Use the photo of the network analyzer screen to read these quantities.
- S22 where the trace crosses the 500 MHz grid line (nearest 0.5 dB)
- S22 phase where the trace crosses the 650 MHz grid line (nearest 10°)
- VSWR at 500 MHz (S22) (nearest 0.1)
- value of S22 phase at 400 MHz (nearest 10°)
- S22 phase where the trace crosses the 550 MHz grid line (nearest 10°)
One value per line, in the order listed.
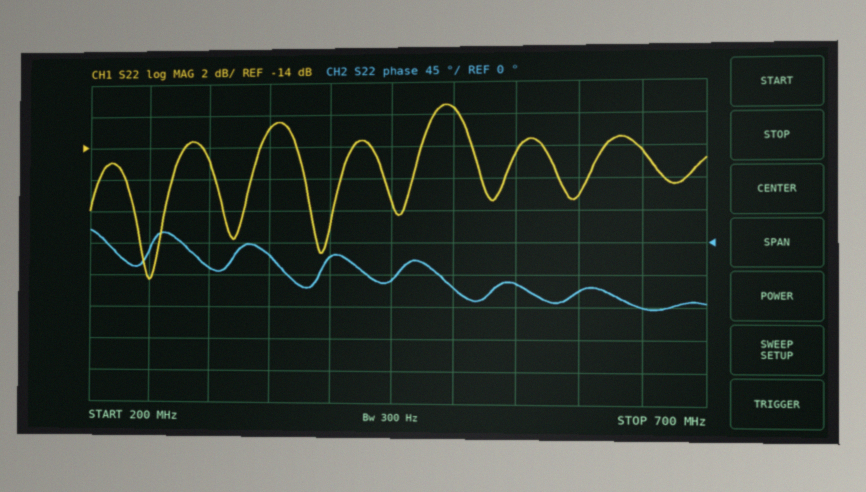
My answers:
-11.5 dB
-90°
1.7
-20°
-60°
